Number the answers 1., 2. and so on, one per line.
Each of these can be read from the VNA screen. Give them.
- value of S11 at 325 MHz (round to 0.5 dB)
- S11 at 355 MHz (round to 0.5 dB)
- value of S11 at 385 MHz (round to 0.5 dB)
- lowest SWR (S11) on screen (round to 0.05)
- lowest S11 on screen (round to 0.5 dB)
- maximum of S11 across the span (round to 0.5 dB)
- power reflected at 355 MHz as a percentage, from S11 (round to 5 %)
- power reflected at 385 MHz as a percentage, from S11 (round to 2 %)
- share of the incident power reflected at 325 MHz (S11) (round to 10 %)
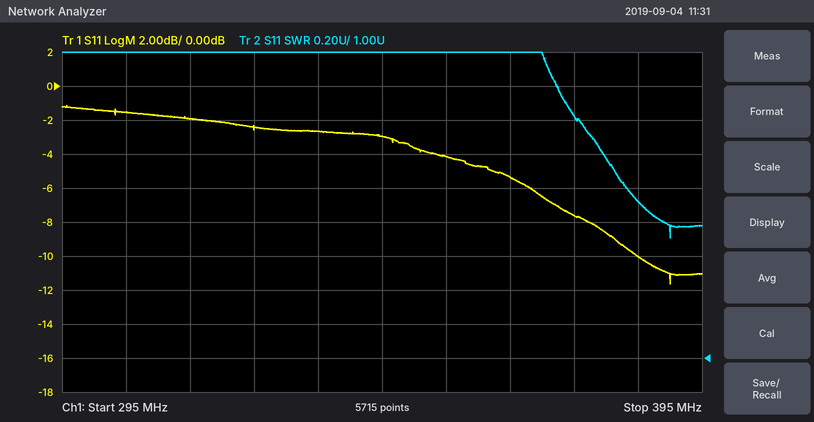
1. -2.5 dB
2. -4.0 dB
3. -10.0 dB
4. 1.70
5. -11.5 dB
6. -1.0 dB
7. 40 %
8. 10 %
9. 60 %
